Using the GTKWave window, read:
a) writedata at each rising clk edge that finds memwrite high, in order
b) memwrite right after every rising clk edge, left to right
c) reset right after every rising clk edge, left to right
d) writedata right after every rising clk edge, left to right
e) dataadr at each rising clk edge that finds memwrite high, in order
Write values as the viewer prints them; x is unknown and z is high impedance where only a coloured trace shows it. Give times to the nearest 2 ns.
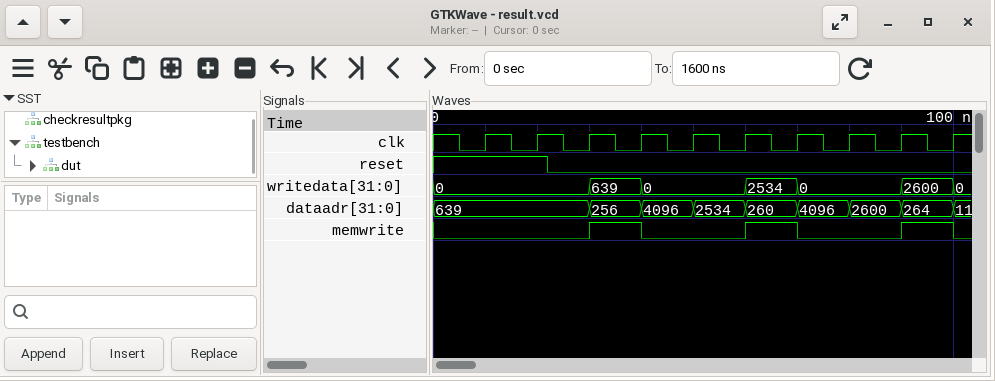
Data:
639, 2534, 2600
0 0 1 0 0 1 0 0 1 0
1 1 0 0 0 0 0 0 0 0
0, 0, 639, 0, 0, 2534, 0, 0, 2600, 0
256, 260, 264
